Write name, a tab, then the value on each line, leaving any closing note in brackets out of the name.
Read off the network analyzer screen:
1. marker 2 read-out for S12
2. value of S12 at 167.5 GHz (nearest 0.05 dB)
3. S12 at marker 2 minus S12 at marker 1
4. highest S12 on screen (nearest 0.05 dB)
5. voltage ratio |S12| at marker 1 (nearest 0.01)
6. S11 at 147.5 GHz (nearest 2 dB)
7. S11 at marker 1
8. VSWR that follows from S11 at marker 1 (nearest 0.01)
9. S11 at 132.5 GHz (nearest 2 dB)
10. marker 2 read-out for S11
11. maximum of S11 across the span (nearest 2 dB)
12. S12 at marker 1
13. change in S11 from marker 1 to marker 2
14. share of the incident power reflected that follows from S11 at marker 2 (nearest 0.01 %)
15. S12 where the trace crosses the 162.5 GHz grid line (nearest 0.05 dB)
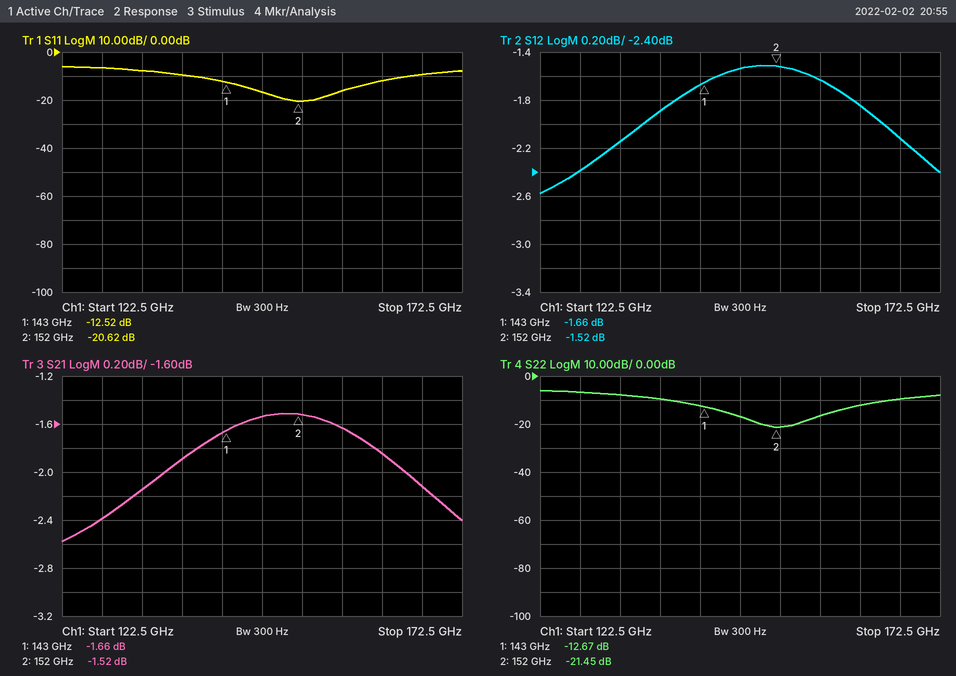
marker 2 read-out for S12	-1.52 dB
value of S12 at 167.5 GHz	-2.10 dB
S12 at marker 2 minus S12 at marker 1	0.14 dB
highest S12 on screen	-1.50 dB
voltage ratio |S12| at marker 1	0.83
S11 at 147.5 GHz	-16 dB
S11 at marker 1	-12.52 dB
VSWR that follows from S11 at marker 1	1.62
S11 at 132.5 GHz	-8 dB
marker 2 read-out for S11	-20.62 dB
maximum of S11 across the span	-6 dB
S12 at marker 1	-1.66 dB
change in S11 from marker 1 to marker 2	-8.10 dB
share of the incident power reflected that follows from S11 at marker 2	0.87 %
S12 where the trace crosses the 162.5 GHz grid line	-1.85 dB
